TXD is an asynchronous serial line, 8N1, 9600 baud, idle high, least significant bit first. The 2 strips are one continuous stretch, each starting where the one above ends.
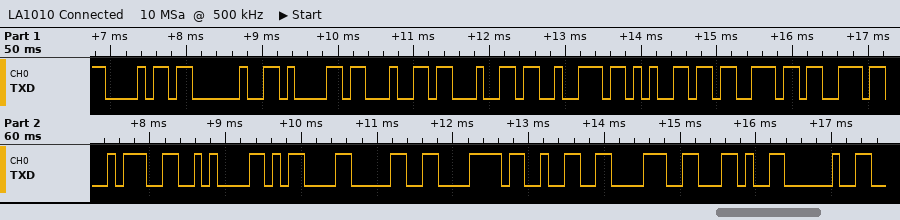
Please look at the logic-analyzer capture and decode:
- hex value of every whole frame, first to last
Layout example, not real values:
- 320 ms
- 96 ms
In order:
- 0x68 0x20 0x61 0x64 0x64 0x72 0x65 0x73 0x73 0x3A 0x0A 0x0D 0x30 0x78 0x32 0x38 0x2C 0x20
